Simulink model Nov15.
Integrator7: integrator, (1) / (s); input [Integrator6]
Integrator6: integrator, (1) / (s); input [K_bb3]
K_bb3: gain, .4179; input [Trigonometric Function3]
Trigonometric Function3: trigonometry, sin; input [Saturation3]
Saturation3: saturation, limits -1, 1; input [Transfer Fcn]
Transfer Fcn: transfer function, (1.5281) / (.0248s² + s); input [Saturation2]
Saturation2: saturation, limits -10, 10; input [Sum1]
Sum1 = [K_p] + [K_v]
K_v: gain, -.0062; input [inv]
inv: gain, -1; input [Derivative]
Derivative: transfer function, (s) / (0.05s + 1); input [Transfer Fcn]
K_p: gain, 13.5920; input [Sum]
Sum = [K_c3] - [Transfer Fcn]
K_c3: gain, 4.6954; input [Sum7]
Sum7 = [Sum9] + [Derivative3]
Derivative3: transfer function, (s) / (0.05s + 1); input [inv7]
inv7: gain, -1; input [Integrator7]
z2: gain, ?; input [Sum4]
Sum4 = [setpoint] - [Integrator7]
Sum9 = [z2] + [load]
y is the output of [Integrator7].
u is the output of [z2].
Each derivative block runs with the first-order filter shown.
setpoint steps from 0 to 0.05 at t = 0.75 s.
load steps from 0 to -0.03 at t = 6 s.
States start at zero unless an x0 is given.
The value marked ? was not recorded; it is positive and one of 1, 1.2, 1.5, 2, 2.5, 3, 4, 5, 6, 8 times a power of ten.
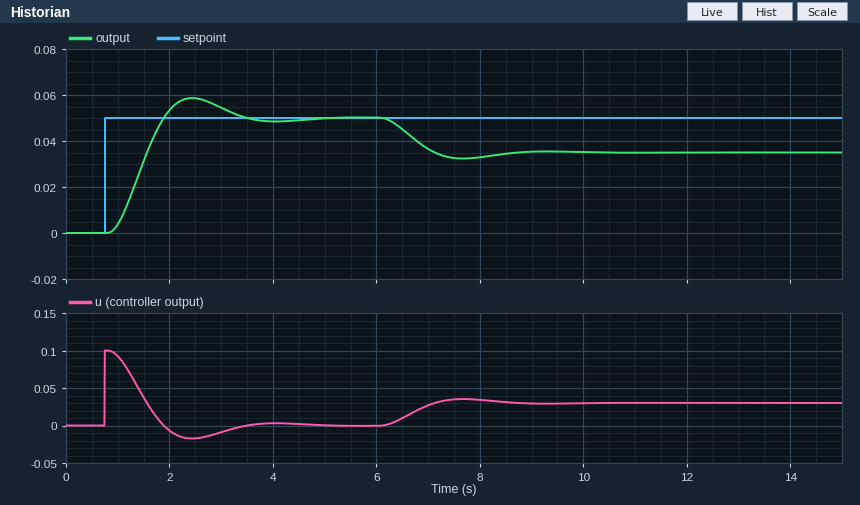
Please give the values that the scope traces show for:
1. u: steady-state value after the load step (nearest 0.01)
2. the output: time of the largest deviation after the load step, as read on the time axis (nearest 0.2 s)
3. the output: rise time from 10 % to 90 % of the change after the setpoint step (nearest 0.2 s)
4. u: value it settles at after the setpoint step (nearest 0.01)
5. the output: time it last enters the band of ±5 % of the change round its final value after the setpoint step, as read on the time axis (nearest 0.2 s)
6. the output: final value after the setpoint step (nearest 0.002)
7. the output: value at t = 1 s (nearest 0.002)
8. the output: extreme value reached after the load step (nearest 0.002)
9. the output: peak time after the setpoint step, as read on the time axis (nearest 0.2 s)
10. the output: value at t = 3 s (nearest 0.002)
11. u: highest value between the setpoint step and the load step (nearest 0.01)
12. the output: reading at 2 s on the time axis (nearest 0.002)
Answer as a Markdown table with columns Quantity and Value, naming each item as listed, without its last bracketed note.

| Quantity | Value |
|---|---|
| u: steady-state value after the load step | 0.03 |
| the output: time of the largest deviation after the load step, as read on the time axis | 7.6 s |
| the output: rise time from 10 % to 90 % of the change after the setpoint step | 0.8 s |
| u: value it settles at after the setpoint step | 0.00 |
| the output: time it last enters the band of ±5 % of the change round its final value after the setpoint step, as read on the time axis | 3.2 s |
| the output: final value after the setpoint step | 0.050 |
| the output: value at t = 1 s | 0.004 |
| the output: extreme value reached after the load step | 0.032 |
| the output: peak time after the setpoint step, as read on the time axis | 2.4 s |
| the output: value at t = 3 s | 0.054 |
| u: highest value between the setpoint step and the load step | 0.10 |
| the output: reading at 2 s on the time axis | 0.054 |
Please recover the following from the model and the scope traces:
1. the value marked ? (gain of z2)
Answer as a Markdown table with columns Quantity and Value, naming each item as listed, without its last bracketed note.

| Quantity | Value |
|---|---|
| the value marked ? | 2 |
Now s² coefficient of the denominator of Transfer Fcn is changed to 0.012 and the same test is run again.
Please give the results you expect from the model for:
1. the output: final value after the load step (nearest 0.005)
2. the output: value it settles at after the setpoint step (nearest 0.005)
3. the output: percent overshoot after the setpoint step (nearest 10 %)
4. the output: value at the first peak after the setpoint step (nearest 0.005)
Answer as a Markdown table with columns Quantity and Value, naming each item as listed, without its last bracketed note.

| Quantity | Value |
|---|---|
| the output: final value after the load step | 0.035 |
| the output: value it settles at after the setpoint step | 0.050 |
| the output: percent overshoot after the setpoint step | 20 % |
| the output: value at the first peak after the setpoint step | 0.060 |
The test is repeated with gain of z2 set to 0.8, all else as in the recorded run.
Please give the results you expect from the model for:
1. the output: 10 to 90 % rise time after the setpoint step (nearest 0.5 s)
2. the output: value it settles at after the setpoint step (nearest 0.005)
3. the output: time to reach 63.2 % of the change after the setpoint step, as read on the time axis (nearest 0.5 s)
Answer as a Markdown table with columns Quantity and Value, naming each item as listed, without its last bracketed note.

| Quantity | Value |
|---|---|
| the output: 10 to 90 % rise time after the setpoint step | 2.0 s |
| the output: value it settles at after the setpoint step | 0.050 |
| the output: time to reach 63.2 % of the change after the setpoint step, as read on the time axis | 2.0 s |
